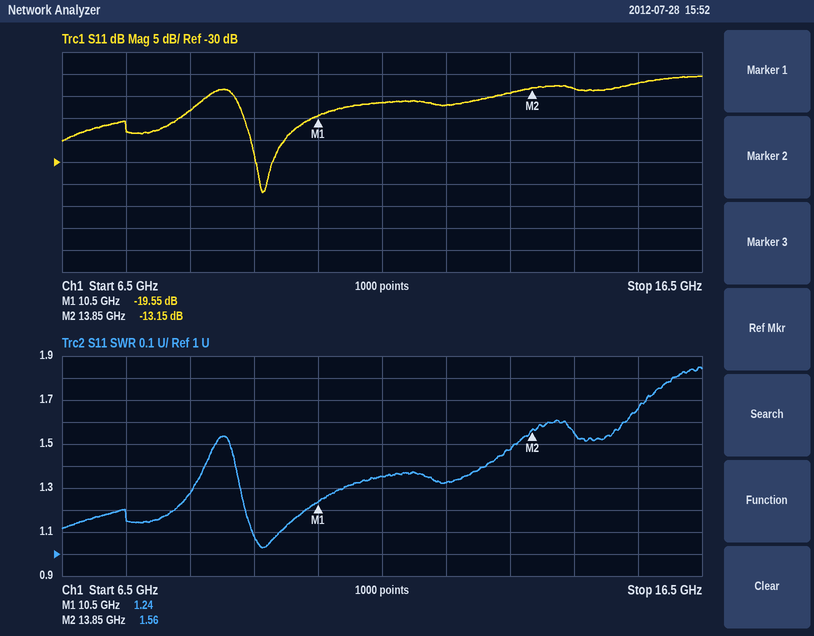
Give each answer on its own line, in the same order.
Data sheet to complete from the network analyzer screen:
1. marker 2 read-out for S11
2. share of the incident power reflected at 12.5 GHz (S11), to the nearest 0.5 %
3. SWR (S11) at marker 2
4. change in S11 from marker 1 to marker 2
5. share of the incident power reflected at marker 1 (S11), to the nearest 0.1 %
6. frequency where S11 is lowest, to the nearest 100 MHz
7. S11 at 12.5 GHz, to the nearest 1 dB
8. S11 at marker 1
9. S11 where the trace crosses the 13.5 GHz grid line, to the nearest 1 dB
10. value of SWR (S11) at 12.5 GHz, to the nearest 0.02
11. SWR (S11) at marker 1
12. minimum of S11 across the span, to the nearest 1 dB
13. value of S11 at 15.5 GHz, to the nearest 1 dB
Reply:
-13.15 dB
2.0 %
1.56
6.40 dB
1.1 %
9.6 GHz
-17 dB
-19.55 dB
-14 dB
1.32
1.24
-37 dB
-12 dB
